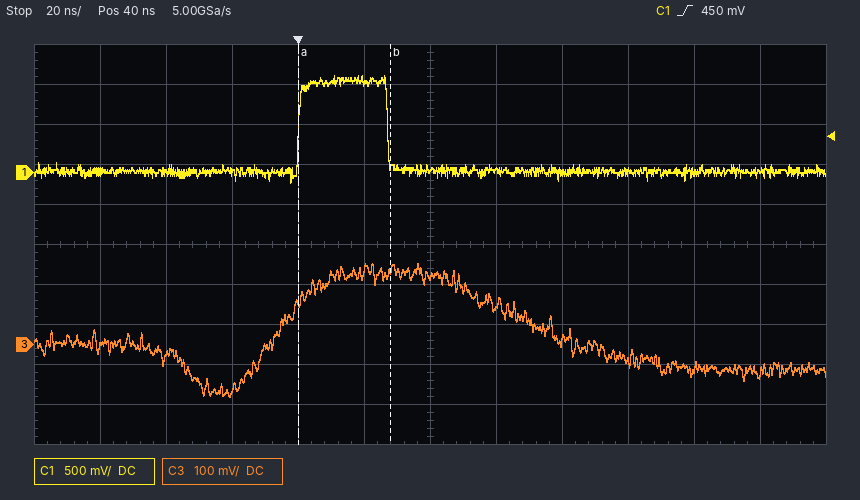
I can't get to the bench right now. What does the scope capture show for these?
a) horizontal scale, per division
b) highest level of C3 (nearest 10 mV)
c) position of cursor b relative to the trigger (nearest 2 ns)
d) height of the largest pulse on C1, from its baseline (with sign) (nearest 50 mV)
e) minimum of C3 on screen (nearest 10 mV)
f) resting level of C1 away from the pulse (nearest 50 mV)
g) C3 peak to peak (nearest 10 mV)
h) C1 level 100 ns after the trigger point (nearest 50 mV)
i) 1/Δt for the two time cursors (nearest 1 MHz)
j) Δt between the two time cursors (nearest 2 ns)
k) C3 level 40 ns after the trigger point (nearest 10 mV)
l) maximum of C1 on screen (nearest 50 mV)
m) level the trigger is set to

20 ns
200 mV
+28 ns
+1.20 V
-130 mV
0 mV
330 mV
0 mV
36 MHz
28 ns
170 mV
1.20 V
450 mV
